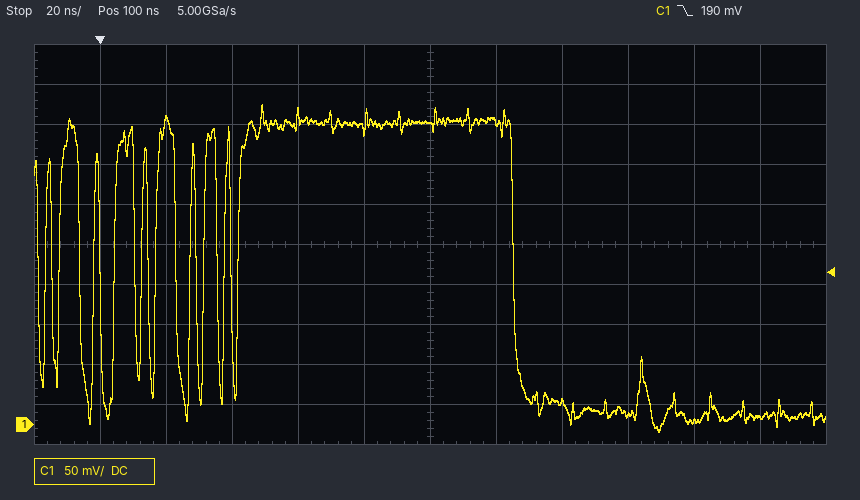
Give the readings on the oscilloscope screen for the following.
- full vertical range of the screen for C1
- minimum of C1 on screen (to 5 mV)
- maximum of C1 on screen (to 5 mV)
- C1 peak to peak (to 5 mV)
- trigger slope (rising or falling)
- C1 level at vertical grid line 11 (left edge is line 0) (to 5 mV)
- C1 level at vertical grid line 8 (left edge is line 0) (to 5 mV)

500 mV
-10 mV
400 mV
410 mV
falling
10 mV
30 mV
